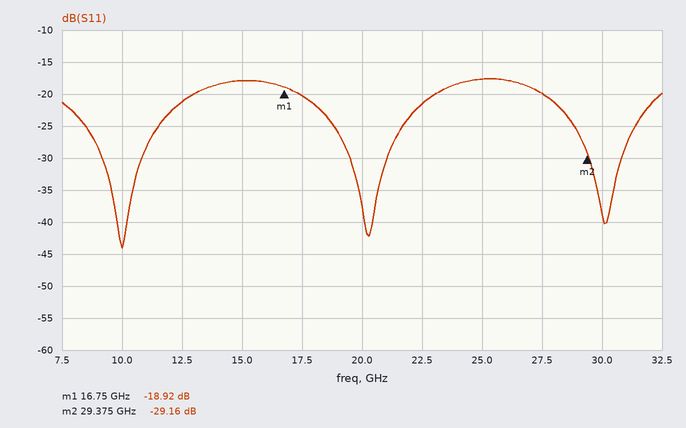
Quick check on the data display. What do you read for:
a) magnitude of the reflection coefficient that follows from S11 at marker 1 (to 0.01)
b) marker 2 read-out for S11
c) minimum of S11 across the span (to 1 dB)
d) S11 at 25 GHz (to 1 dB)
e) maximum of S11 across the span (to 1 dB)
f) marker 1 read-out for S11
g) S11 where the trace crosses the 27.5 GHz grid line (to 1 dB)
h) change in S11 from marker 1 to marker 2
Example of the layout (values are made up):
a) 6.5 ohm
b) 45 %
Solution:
a) 0.11
b) -29.16 dB
c) -44 dB
d) -18 dB
e) -18 dB
f) -18.92 dB
g) -20 dB
h) -10.24 dB
